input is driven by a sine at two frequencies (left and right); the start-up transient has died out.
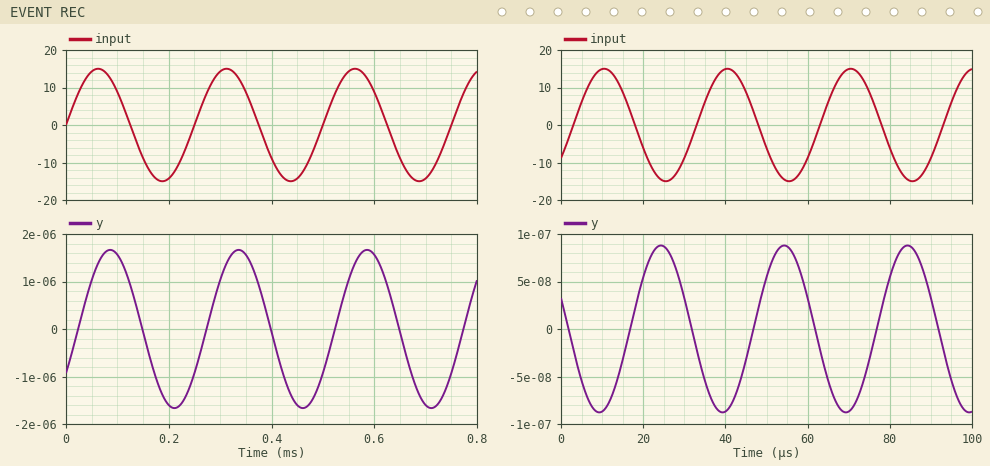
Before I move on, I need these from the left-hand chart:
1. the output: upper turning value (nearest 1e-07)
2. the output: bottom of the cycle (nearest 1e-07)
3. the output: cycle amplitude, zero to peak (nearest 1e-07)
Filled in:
0.0000017
-0.0000017
0.0000017
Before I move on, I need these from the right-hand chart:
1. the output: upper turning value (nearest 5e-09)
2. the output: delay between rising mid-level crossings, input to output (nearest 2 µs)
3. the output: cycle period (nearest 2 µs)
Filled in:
0.000000090
14 µs
30 µs
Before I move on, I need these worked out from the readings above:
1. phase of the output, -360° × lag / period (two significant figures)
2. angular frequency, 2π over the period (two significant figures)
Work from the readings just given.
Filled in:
-170°
0.21 rad/µs
